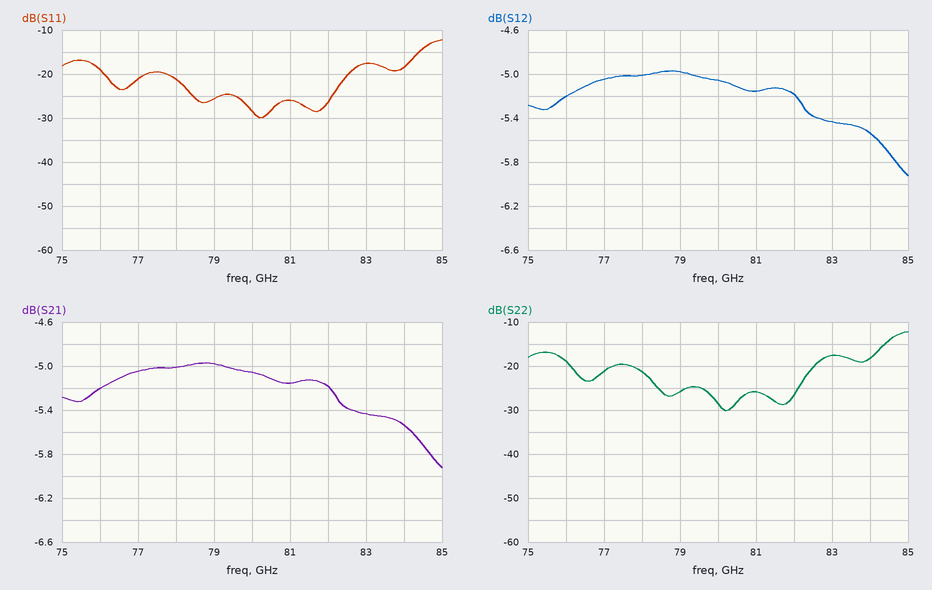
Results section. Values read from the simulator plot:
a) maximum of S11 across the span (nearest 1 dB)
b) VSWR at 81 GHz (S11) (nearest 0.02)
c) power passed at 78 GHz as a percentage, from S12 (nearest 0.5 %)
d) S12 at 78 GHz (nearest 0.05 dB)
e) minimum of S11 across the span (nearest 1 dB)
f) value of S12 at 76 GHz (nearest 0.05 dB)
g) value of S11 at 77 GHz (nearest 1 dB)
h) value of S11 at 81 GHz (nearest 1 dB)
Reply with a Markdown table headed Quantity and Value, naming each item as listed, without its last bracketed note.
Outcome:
| Quantity | Value |
|---|---|
| maximum of S11 across the span | -12 dB |
| VSWR at 81 GHz (S11) | 1.10 |
| power passed at 78 GHz as a percentage, from S12 | 31.5 % |
| S12 at 78 GHz | -5.00 dB |
| minimum of S11 across the span | -30 dB |
| value of S12 at 76 GHz | -5.20 dB |
| value of S11 at 77 GHz | -21 dB |
| value of S11 at 81 GHz | -26 dB |
